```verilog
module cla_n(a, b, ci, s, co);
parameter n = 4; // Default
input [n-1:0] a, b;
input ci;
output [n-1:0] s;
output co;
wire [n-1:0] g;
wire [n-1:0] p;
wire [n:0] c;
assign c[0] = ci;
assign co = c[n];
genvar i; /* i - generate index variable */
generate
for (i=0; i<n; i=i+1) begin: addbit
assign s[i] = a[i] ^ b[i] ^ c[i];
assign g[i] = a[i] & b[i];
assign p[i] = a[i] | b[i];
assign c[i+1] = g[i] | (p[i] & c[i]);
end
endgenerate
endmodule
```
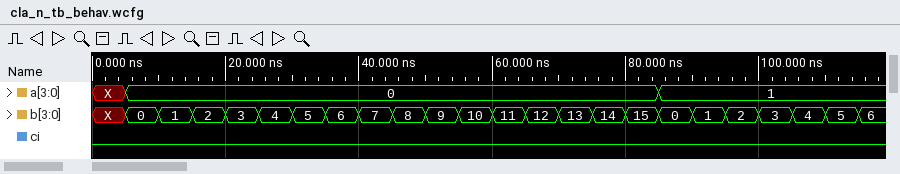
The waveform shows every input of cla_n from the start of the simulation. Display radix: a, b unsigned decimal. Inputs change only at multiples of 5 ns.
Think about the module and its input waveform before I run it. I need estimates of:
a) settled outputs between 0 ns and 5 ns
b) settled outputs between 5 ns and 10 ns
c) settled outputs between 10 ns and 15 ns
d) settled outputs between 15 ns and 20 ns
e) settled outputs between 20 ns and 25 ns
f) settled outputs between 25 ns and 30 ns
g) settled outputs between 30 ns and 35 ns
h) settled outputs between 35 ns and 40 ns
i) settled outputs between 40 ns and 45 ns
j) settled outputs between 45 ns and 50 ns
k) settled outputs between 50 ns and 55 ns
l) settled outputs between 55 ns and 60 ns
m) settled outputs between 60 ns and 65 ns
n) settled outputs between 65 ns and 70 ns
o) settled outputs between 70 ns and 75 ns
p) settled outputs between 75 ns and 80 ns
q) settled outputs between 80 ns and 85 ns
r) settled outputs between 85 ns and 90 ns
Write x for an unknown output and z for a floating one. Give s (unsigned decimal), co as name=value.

s=x, co=x
s=0, co=0
s=1, co=0
s=2, co=0
s=3, co=0
s=4, co=0
s=5, co=0
s=6, co=0
s=7, co=0
s=8, co=0
s=9, co=0
s=10, co=0
s=11, co=0
s=12, co=0
s=13, co=0
s=14, co=0
s=15, co=0
s=1, co=0
